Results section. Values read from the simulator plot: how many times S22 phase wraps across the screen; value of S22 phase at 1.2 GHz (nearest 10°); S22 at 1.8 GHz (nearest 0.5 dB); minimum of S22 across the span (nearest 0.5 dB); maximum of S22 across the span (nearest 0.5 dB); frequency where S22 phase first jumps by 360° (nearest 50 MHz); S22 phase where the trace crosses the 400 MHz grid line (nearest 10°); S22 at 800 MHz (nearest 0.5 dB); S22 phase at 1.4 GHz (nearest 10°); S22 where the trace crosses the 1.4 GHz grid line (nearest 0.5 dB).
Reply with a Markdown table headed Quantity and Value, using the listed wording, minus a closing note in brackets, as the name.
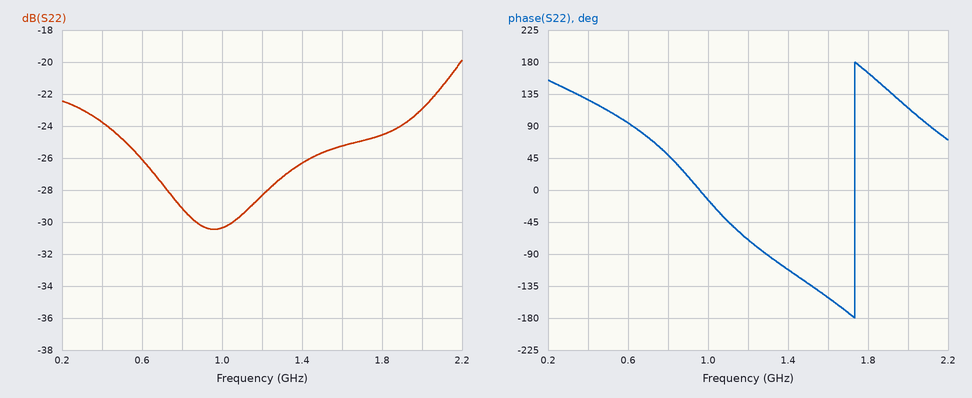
| Quantity | Value |
|---|---|
| how many times S22 phase wraps across the screen | 1 |
| value of S22 phase at 1.2 GHz | -70° |
| S22 at 1.8 GHz | -24.5 dB |
| minimum of S22 across the span | -30.5 dB |
| maximum of S22 across the span | -20.0 dB |
| frequency where S22 phase first jumps by 360° | 1.75 GHz |
| S22 phase where the trace crosses the 400 MHz grid line | 130° |
| S22 at 800 MHz | -29.0 dB |
| S22 phase at 1.4 GHz | -110° |
| S22 where the trace crosses the 1.4 GHz grid line | -26.5 dB |
